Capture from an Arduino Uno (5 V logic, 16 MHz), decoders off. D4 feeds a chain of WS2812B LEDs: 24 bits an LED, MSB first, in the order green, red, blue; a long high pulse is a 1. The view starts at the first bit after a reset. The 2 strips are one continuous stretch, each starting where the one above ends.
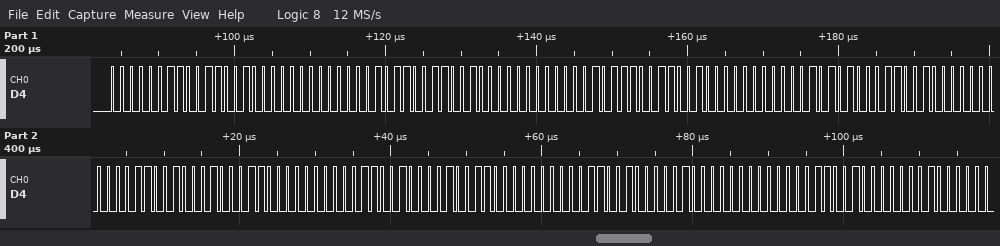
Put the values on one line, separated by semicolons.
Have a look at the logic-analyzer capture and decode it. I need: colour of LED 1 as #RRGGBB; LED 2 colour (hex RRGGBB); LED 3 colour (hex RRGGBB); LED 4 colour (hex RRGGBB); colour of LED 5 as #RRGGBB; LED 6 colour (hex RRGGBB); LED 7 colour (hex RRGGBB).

#320300; #320B00; #321700; #322A00; #233200; #133200; #083200
